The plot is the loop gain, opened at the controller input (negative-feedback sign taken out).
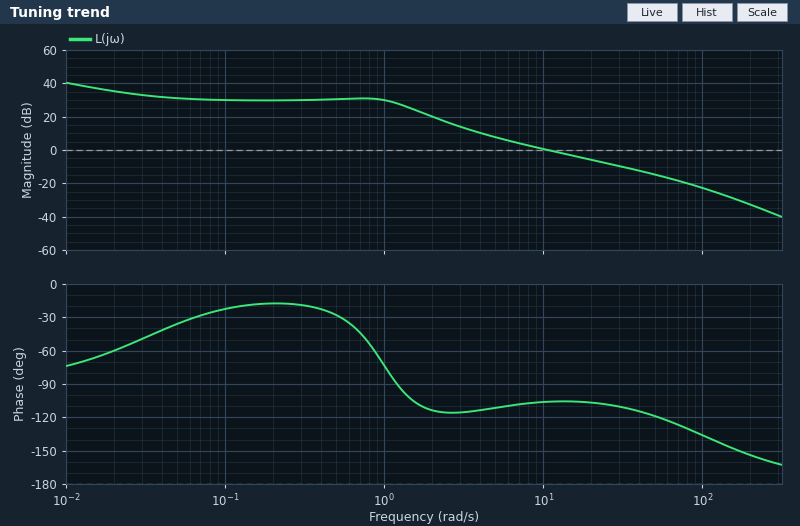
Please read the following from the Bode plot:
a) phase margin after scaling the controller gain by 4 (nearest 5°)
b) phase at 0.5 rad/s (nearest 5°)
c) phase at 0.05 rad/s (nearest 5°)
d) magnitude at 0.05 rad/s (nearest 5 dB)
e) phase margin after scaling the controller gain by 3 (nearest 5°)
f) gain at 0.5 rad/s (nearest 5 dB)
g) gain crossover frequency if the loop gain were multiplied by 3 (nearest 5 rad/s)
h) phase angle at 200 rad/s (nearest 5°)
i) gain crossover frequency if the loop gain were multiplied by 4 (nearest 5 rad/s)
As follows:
65°
-30°
-35°
30 dB
70°
30 dB
30 rad/s
-155°
40 rad/s
